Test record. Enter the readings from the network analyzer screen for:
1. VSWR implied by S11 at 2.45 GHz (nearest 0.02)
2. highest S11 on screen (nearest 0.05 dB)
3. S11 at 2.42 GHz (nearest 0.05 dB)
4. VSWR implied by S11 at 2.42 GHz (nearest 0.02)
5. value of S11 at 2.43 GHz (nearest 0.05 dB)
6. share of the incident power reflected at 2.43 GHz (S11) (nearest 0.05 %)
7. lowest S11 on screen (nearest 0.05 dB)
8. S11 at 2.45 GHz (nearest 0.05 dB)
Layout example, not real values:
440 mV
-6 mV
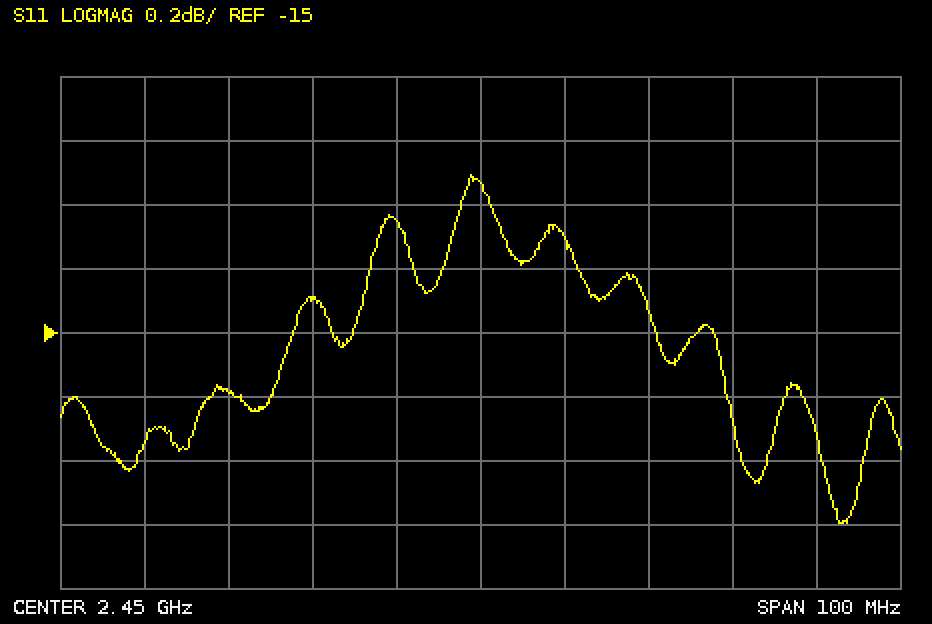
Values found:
1.46
-14.50 dB
-15.20 dB
1.42
-14.90 dB
3.25 %
-15.60 dB
-14.55 dB
